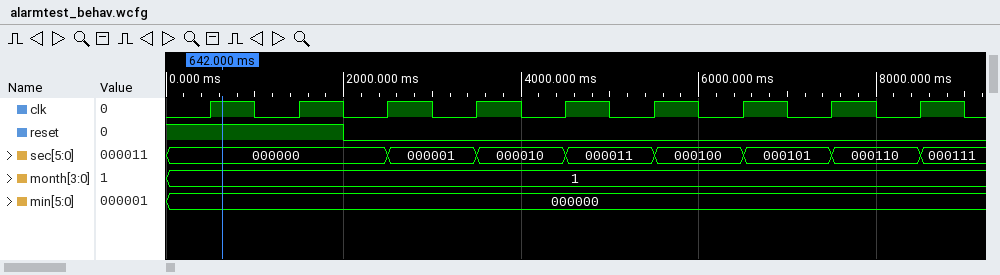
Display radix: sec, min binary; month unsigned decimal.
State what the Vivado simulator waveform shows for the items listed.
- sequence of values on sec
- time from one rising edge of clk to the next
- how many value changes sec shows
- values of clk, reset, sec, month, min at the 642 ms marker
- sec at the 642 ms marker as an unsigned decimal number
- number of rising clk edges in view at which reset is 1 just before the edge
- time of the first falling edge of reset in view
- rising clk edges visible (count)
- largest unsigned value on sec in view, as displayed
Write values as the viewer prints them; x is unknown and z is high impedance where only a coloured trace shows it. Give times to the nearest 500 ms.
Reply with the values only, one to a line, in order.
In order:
000000, 000001, 000010, 000011, 000100, 000101, 000110, 000111
1000 ms
7
clk=1, reset=1, sec=000000, month=1, min=000000
0
2
2000 ms
9
000111
